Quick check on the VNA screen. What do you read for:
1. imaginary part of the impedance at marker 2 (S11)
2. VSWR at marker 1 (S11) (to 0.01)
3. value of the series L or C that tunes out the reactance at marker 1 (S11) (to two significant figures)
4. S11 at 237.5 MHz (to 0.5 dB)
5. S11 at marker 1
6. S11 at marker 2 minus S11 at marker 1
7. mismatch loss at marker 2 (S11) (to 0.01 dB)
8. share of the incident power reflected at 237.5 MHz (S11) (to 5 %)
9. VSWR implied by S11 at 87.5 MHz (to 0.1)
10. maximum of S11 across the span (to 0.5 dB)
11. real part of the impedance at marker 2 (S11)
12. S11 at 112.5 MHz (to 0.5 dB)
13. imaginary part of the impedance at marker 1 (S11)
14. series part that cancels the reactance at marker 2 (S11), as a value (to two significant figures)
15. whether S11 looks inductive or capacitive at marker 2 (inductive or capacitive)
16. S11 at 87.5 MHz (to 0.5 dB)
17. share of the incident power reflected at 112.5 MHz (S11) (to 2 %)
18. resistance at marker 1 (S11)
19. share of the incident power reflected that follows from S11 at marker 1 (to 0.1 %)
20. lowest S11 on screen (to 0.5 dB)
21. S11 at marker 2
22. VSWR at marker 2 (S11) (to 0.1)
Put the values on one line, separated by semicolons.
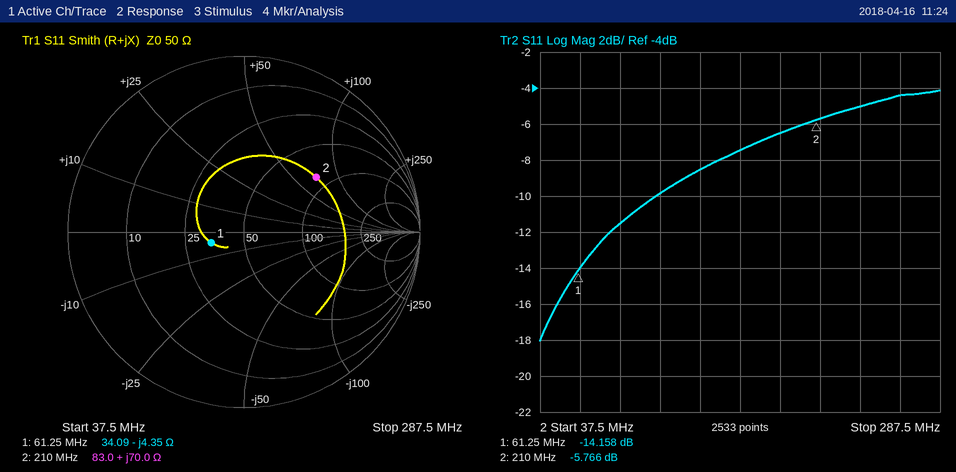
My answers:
+70.0 Ω; 1.49; 11 nH; -5.0 dB; -14.158 dB; 8.392 dB; 1.34 dB; 30 %; 1.7; -4.0 dB; 83.0 Ω; -10.0 dB; -4.35 Ω; 11 pF; inductive; -11.5 dB; 10 %; 34.09 Ω; 3.8 %; -18.0 dB; -5.766 dB; 3.1
